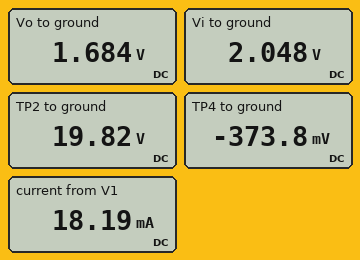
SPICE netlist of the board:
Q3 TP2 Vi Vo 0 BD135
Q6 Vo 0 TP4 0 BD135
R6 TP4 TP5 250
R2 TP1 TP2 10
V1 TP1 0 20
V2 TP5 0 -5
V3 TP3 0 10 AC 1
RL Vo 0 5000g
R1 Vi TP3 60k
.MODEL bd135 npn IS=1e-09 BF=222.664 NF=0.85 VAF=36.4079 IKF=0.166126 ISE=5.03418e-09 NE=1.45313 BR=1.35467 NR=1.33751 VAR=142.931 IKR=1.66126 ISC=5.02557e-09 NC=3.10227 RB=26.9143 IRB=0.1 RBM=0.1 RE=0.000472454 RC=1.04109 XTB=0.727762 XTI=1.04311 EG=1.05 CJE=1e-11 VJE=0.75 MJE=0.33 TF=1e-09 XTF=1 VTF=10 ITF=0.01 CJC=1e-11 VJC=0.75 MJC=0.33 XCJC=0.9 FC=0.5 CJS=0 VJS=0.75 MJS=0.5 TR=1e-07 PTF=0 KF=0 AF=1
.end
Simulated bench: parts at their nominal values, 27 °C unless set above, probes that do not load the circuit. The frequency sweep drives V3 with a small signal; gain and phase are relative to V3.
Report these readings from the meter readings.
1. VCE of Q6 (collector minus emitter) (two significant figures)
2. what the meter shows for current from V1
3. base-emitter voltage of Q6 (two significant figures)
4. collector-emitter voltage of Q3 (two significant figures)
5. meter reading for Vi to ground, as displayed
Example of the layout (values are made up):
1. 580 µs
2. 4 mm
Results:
1. 2.1 V
2. 18.19 mA
3. 370 mV
4. 18 V
5. 2.048 V
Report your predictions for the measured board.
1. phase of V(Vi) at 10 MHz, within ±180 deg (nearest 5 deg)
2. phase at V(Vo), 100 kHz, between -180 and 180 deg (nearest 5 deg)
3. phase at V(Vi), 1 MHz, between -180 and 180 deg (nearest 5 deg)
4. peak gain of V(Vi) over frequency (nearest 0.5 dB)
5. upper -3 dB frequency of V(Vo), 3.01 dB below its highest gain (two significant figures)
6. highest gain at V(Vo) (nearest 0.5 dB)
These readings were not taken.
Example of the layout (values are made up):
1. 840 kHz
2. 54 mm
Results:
1. -95 deg
2. -5 deg
3. -50 deg
4. -1.0 dB
5. 820 kHz
6. -1.0 dB
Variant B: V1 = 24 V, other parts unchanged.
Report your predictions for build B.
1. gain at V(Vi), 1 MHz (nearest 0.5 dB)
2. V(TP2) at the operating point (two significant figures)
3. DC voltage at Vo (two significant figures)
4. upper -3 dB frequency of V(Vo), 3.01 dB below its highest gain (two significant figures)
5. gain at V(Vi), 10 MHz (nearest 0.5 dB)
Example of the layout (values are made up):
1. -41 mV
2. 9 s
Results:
1. -4.5 dB
2. 24 V
3. 2.1 V
4. 870 kHz
5. -22.5 dB
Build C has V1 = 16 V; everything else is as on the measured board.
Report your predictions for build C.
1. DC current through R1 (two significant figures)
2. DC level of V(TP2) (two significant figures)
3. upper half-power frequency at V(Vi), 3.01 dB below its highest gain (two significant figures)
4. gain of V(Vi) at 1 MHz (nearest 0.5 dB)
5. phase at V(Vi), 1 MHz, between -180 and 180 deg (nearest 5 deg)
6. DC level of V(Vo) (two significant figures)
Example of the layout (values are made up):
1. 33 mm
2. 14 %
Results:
1. 140 µA
2. 16 V
3. 770 kHz
4. -5.5 dB
5. -55 deg
6. 1.2 V
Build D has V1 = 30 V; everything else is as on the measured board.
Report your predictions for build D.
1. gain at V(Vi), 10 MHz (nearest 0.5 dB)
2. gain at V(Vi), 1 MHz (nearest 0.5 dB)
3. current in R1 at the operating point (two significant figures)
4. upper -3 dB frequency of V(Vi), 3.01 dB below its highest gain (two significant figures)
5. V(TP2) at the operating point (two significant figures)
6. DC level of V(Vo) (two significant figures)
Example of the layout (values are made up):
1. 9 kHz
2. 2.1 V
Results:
1. -21.5 dB
2. -4.0 dB
3. 120 µA
4. 930 kHz
5. 30 V
6. 2.6 V
